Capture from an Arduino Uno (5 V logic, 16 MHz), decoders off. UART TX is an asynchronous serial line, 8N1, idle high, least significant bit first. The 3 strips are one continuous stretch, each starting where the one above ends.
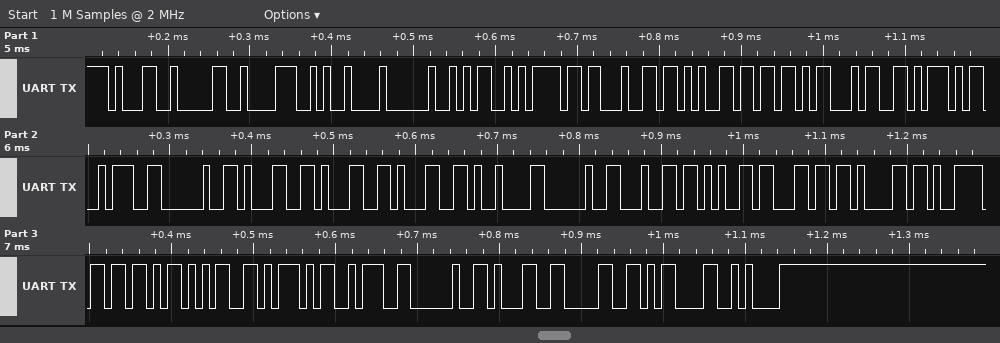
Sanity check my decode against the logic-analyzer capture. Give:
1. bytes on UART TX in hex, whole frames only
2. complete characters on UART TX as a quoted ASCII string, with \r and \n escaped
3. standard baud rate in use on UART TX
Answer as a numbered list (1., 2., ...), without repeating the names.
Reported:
1. 0x31 0x30 0x38 0x09 0x20 0x4D 0x6F 0x64 0x65 0x5B 0x34 0x5D 0x3A 0x20 0x31 0x31 0x31 0x09 0x20 0x64 0x65 0x6C 0x61 0x79 0x5B 0x35 0x5D 0x3A 0x20 0x31 0x30 0x0D 0x0A
2. "108\t Mode[4]: 111\t delay[5]: 10\r\n"
3. 115200 baud
